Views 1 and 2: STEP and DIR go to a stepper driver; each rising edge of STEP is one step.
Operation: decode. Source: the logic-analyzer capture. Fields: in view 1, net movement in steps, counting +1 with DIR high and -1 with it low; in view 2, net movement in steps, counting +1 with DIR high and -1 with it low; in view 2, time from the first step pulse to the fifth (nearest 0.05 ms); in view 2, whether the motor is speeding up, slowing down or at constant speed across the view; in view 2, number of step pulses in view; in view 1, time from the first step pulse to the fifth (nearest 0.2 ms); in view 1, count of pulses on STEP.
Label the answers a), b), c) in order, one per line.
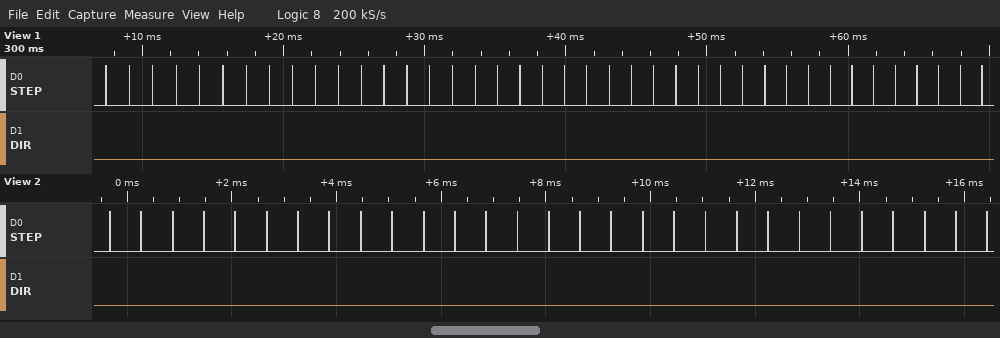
a) -40
b) -29
c) 2.40 ms
d) constant speed
e) 29
f) 6.6 ms
g) 40
